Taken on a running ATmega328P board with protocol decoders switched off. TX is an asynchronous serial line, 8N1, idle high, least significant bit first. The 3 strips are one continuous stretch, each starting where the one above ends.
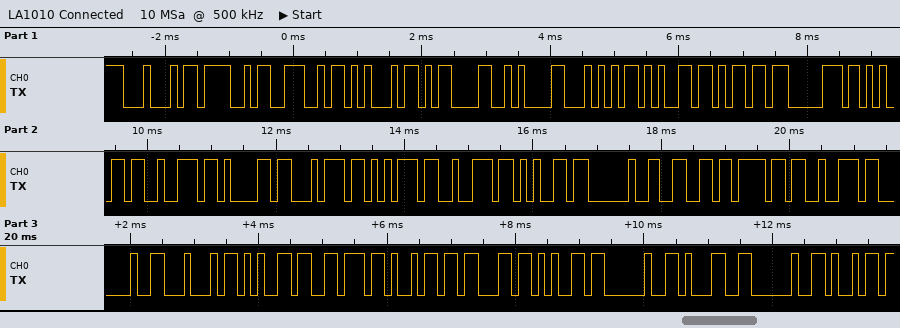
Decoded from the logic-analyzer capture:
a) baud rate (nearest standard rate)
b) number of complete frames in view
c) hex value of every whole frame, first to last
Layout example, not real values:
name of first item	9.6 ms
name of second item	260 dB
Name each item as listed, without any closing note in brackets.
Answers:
baud rate	9600 baud
number of complete frames in view	32
hex value of every whole frame, first to last	44 4F 4E 45 0D 0A 54 65 6D 70 65 72 61 74 75 72 65 20 66 6F 72 20 44 65 76 69 63 65 20 31 20 69
